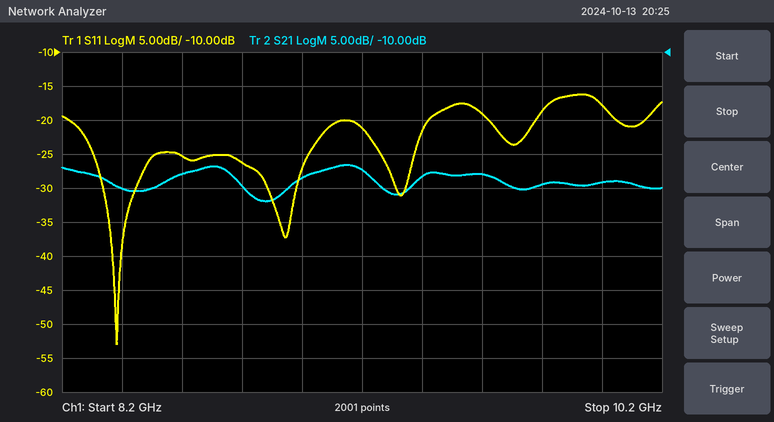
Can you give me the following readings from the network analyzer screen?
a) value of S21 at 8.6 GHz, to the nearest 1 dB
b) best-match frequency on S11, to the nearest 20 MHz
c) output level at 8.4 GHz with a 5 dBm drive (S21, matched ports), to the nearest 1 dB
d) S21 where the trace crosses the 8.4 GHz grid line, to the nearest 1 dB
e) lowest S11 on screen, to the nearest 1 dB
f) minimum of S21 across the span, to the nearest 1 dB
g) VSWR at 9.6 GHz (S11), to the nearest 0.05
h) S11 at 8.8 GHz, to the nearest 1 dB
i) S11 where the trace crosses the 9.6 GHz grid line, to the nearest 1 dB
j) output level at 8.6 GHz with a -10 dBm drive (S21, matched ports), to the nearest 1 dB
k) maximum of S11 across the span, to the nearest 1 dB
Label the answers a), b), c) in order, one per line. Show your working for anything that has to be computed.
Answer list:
a) -28 dB
b) 8.38 GHz
c) 5 dBm + (-30 dB) = -25 dBm
d) -30 dB
e) -53 dB
f) -32 dB
g) |Γ| = 10^(-19/20) = 0.1122; VSWR = (1 + 0.1122)/(1 − 0.1122) ≈ 1.25
h) -26 dB
i) -19 dB
j) -10 dBm + (-28 dB) = -38 dBm
k) -16 dB
